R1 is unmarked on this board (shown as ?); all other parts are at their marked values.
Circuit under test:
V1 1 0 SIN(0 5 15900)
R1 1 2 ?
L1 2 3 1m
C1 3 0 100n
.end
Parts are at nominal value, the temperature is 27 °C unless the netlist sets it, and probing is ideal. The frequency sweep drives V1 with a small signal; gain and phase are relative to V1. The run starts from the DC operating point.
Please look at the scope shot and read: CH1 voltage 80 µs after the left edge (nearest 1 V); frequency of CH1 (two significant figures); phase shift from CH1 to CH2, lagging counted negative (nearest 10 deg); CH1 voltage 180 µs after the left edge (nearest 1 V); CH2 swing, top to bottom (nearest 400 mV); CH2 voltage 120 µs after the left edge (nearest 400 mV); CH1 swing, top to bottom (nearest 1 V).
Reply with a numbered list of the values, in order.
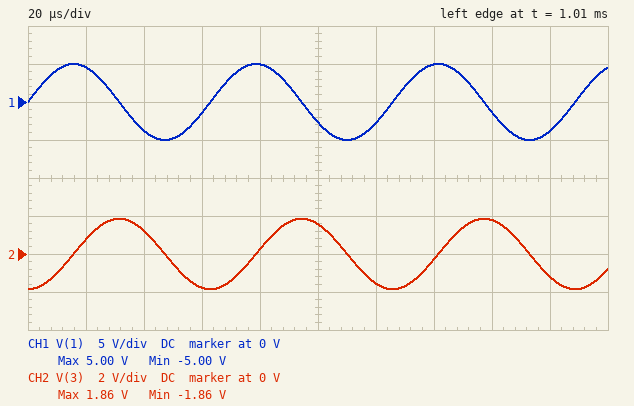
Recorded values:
1. 5 V
2. 16 kHz
3. -90 deg
4. -4 V
5. 3.6 V
6. -1.6 V
7. 10 V
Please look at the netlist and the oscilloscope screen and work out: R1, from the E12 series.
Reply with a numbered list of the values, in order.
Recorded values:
1. 270 Ω
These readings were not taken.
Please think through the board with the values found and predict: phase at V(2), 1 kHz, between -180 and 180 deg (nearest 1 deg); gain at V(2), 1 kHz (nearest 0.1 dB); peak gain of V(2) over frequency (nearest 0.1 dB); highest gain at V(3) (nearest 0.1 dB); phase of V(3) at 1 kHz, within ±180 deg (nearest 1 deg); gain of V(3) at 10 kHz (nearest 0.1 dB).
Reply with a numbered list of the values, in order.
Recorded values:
1. -10 deg
2. -0.1 dB
3. 0 dB
4. 0 dB
5. -10 deg
6. -5.1 dB
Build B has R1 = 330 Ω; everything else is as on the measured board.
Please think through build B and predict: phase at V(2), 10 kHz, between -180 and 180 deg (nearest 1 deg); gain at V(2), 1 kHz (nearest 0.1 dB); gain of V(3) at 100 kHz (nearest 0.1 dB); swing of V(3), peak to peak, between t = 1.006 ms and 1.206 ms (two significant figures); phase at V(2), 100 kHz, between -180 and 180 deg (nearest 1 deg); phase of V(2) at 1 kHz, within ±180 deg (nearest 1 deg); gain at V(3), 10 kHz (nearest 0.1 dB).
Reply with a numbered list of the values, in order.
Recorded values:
1. -74 deg
2. -0.2 dB
3. -32.8 dB
4. 3.0 V
5. 28 deg
6. -12 deg
7. -6.7 dB
